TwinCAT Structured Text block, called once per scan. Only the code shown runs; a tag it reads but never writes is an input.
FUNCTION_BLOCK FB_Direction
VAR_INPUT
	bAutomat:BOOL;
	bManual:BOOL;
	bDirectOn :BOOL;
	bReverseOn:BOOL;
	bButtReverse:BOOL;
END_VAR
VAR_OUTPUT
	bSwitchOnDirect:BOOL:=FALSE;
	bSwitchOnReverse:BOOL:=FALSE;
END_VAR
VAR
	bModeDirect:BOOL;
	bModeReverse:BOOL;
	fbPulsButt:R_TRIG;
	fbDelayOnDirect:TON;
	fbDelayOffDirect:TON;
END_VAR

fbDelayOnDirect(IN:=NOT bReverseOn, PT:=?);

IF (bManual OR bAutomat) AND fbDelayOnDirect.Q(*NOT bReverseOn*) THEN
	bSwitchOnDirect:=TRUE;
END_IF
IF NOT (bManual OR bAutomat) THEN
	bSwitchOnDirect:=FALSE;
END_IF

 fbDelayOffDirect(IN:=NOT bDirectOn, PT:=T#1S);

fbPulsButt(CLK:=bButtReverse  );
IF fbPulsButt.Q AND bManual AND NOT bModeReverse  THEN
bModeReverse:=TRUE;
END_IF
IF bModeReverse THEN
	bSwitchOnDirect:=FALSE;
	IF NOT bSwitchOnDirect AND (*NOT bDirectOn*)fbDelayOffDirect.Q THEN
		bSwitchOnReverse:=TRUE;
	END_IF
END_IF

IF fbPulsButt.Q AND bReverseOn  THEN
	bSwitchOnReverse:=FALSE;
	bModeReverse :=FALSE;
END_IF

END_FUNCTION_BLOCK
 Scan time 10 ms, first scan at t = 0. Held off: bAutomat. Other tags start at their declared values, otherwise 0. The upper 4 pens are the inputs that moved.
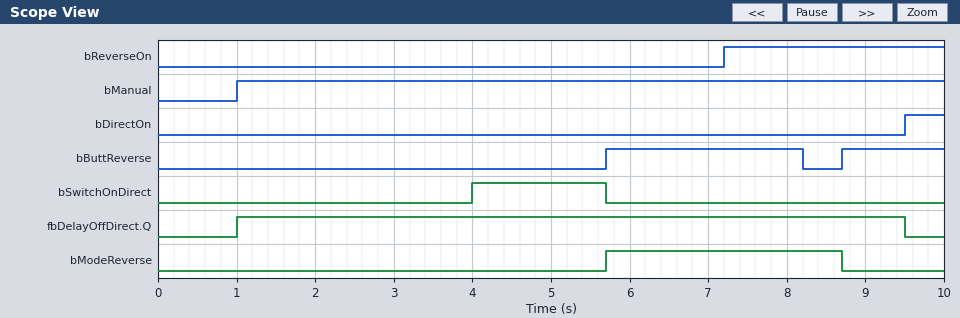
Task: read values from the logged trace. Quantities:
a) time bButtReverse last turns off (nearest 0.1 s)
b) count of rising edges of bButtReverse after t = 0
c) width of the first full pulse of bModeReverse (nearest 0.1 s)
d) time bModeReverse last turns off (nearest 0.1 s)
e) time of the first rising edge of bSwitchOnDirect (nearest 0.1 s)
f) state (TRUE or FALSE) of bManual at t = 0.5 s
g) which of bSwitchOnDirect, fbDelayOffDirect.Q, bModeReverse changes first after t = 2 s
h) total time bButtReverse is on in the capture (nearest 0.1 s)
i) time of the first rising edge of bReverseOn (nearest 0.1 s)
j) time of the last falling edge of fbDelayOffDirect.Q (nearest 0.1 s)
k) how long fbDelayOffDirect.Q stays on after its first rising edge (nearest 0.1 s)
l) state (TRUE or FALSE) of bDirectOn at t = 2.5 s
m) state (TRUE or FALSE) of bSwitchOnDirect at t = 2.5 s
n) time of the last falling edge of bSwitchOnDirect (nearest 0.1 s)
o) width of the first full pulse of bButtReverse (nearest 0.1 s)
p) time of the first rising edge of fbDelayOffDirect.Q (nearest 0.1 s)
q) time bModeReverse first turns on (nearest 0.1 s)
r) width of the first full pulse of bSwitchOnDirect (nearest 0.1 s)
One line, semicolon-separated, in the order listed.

8.2 s; 2; 3.0 s; 8.7 s; 4.0 s; FALSE; bSwitchOnDirect; 3.8 s; 7.2 s; 9.5 s; 8.5 s; FALSE; FALSE; 5.7 s; 2.5 s; 1.0 s; 5.7 s; 1.7 s
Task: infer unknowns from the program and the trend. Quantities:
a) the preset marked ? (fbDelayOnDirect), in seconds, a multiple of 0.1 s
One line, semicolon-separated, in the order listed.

4.0 s
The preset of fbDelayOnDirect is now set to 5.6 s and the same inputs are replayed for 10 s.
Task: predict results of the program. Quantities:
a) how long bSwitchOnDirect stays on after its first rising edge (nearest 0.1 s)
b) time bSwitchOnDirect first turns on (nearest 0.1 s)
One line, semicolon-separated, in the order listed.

0.1 s; 5.6 s
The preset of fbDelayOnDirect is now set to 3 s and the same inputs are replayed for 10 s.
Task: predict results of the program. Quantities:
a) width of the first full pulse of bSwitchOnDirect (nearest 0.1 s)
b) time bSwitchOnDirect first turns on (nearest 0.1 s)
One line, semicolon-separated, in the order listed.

2.7 s; 3.0 s
